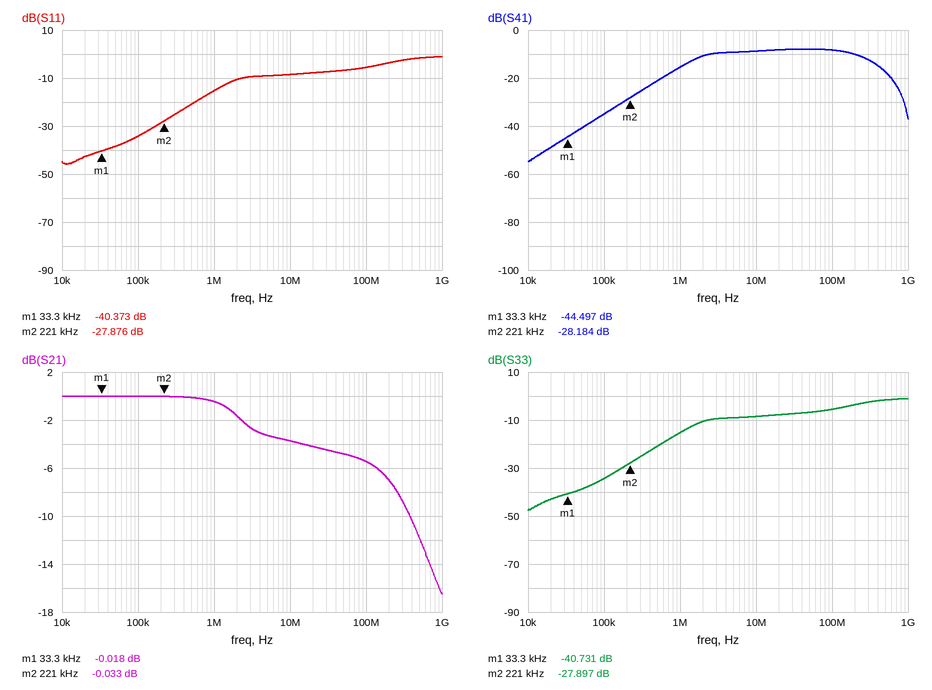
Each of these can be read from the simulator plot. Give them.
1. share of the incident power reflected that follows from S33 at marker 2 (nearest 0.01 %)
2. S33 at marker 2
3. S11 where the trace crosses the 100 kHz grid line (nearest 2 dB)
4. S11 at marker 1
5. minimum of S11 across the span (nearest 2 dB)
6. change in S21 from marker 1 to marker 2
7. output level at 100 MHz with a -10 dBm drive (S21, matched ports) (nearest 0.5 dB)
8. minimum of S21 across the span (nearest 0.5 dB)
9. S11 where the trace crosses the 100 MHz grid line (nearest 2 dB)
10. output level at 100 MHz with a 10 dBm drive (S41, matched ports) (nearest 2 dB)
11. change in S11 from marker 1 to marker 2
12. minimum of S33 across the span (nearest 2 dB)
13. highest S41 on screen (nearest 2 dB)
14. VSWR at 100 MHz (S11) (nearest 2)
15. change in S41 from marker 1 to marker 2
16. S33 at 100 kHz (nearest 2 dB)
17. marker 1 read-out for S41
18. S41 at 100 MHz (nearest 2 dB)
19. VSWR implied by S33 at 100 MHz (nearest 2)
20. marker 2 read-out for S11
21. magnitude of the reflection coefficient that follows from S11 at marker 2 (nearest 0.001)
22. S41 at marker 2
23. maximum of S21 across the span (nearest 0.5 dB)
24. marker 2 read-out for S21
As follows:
0.16 %
-27.897 dB
-34 dB
-40.373 dB
-46 dB
-0.015 dB
-15.5 dBm
-16.5 dB
-6 dB
2 dBm
12.497 dB
-48 dB
-8 dB
4
16.313 dB
-34 dB
-44.497 dB
-8 dB
4
-27.876 dB
0.040
-28.184 dB
0.0 dB
-0.033 dB
